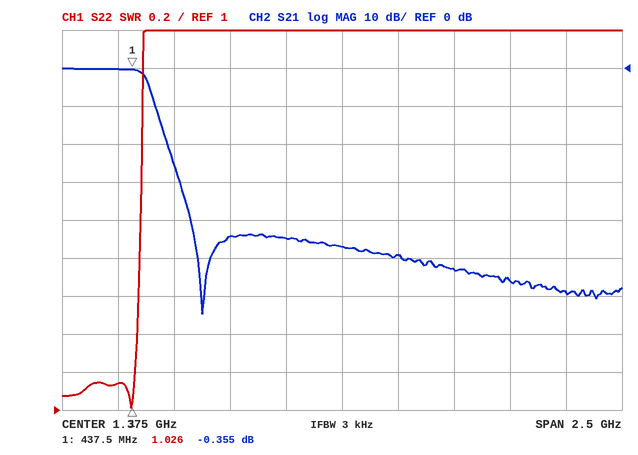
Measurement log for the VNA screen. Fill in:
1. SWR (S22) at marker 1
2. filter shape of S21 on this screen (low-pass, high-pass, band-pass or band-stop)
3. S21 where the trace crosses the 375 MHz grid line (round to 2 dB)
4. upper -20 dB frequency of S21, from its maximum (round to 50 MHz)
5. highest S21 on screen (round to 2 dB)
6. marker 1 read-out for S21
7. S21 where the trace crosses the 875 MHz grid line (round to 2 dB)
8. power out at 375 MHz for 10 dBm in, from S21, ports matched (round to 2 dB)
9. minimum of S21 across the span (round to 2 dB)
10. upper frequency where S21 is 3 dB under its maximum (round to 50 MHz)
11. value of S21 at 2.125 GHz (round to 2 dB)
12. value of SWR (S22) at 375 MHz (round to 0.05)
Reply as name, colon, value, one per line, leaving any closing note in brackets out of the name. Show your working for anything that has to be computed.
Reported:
SWR (S22) at marker 1: 1.026
filter shape of S21 on this screen: low-pass
S21 where the trace crosses the 375 MHz grid line: 0 dB
upper -20 dB frequency of S21, from its maximum: 600 MHz
highest S21 on screen: 0 dB
marker 1 read-out for S21: -0.355 dB
S21 where the trace crosses the 875 MHz grid line: -44 dB
power out at 375 MHz for 10 dBm in, from S21, ports matched: 10 dBm + (0 dB) = 10 dBm
minimum of S21 across the span: -64 dB
upper frequency where S21 is 3 dB under its maximum: 500 MHz
value of S21 at 2.125 GHz: -56 dB
value of SWR (S22) at 375 MHz: 1.15
